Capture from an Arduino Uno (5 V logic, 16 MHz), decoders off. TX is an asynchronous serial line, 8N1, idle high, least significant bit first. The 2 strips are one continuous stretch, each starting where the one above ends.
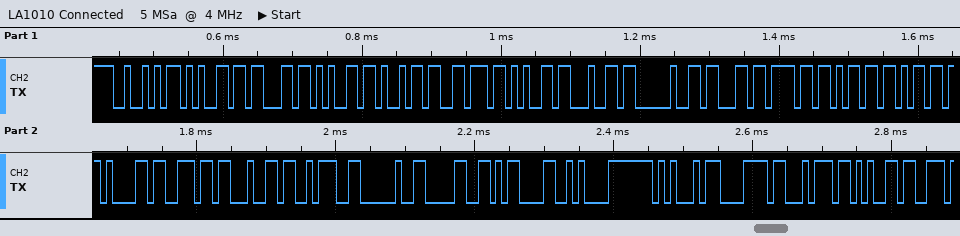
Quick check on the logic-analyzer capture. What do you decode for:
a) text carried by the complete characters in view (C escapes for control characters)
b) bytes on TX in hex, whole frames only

"Received command: 0\r\nExte"
52 65 63 65 69 76 65 64 20 63 6F 6D 6D 61 6E 64 3A 20 30 0D 0A 45 78 74 65
